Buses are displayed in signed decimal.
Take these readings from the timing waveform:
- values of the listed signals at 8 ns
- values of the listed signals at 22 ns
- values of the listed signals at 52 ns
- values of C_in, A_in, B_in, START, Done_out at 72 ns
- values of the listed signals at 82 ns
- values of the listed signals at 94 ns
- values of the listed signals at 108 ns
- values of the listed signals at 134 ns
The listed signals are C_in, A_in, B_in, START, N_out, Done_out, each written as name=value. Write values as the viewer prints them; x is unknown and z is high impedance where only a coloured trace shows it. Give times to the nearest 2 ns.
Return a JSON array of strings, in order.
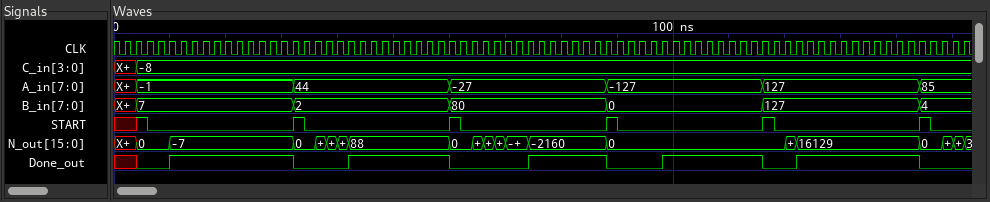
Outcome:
["C_in=-8, A_in=-1, B_in=7, START=0, N_out=0, Done_out=0", "C_in=-8, A_in=-1, B_in=7, START=0, N_out=-7, Done_out=1", "C_in=-8, A_in=44, B_in=2, START=0, N_out=88, Done_out=1", "C_in=-8, A_in=-27, B_in=80, START=0, Done_out=0", "C_in=-8, A_in=-27, B_in=80, START=0, N_out=-2160, Done_out=1", "C_in=-8, A_in=-127, B_in=0, START=0, N_out=0, Done_out=0", "C_in=-8, A_in=-127, B_in=0, START=0, N_out=0, Done_out=1", "C_in=-8, A_in=127, B_in=127, START=0, N_out=16129, Done_out=1"]
